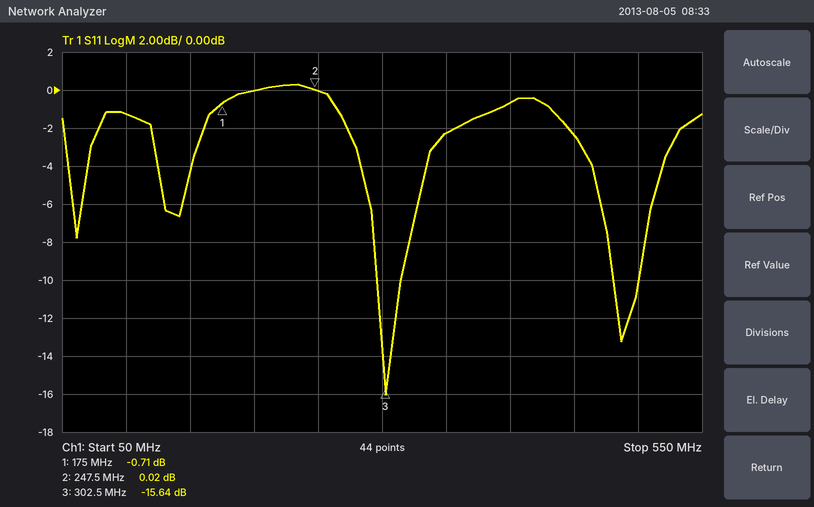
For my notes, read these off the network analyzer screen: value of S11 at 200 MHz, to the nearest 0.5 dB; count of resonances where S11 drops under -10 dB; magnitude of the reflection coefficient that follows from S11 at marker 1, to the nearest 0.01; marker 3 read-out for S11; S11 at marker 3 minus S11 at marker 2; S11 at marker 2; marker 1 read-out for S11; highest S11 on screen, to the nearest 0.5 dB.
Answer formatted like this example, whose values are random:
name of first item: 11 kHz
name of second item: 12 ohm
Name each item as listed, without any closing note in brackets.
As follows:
value of S11 at 200 MHz, to the nearest 0.5 dB: 0.0 dB
count of resonances where S11 drops under -10 dB: 2
magnitude of the reflection coefficient that follows from S11 at marker 1, to the nearest 0.01: 0.92
marker 3 read-out for S11: -15.64 dB
S11 at marker 3 minus S11 at marker 2: -15.66 dB
S11 at marker 2: 0.02 dB
marker 1 read-out for S11: -0.71 dB
highest S11 on screen, to the nearest 0.5 dB: 0.5 dB
